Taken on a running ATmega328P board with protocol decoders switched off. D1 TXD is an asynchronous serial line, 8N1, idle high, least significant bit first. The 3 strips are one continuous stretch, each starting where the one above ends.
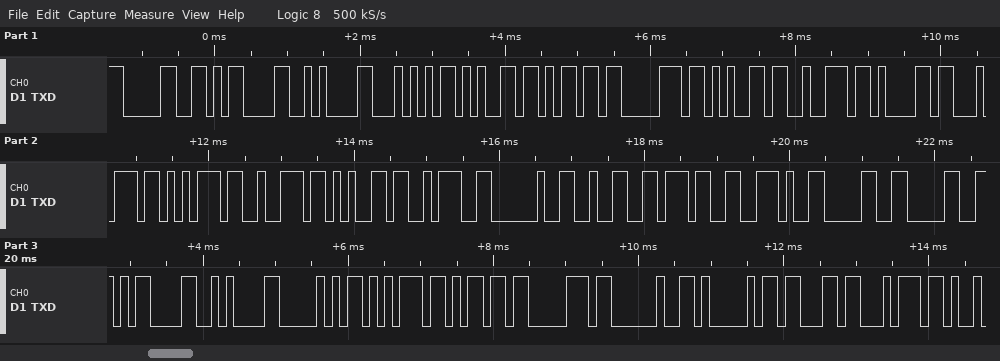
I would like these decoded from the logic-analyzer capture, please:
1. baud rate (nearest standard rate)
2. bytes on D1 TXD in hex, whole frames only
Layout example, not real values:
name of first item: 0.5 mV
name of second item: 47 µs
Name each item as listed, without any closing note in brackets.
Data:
baud rate: 9600 baud
bytes on D1 TXD in hex, whole frames only: 30 0D 0A 54 65 6D 70 65 72 61 74 75 72 65 3A 20 32 37 2E 30 30 0D 0A 50 75 6D 70 20 41 63 74
